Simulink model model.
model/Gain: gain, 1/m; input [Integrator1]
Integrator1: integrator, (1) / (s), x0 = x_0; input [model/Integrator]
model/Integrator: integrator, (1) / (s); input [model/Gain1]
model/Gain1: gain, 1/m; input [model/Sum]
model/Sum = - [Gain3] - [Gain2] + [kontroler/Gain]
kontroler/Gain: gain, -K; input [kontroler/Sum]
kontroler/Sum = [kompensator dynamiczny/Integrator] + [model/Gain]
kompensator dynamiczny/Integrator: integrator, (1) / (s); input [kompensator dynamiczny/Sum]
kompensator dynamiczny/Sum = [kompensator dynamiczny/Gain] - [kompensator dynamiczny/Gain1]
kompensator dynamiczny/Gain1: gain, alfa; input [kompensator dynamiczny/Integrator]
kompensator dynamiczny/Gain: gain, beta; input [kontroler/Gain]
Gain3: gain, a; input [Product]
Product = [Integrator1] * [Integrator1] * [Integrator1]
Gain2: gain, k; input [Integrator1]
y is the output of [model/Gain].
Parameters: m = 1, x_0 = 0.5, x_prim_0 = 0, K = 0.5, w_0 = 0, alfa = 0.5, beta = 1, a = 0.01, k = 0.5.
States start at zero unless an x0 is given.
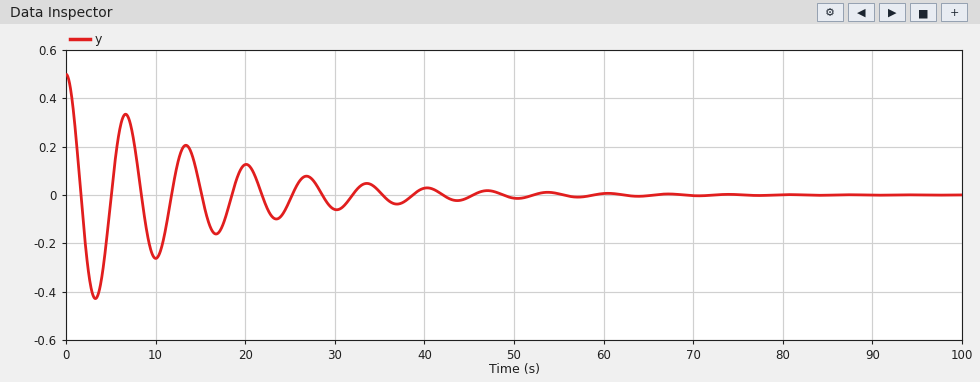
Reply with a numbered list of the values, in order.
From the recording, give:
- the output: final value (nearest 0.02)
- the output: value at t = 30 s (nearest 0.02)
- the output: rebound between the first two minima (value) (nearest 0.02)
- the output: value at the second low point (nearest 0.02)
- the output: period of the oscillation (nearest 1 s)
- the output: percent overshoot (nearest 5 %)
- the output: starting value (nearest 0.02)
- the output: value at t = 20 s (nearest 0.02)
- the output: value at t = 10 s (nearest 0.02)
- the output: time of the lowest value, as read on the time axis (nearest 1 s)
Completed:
1. 0.00
2. -0.06
3. 0.34
4. -0.26
5. 7 s
6. 85 %
7. 0.50
8. 0.12
9. -0.26
10. 3 s
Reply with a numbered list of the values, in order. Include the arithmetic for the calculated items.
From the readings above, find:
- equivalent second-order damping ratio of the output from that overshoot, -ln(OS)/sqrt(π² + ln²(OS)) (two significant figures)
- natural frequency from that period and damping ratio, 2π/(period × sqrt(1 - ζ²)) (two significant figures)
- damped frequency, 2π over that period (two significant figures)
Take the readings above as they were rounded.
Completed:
1. ln(0.85) = -0.163; 0.163 / sqrt(9.870 + 0.026) = 0.052
2. 2π / (7 × sqrt(1 - 0.052²)) = 0.90 rad/s
3. 2π / 7 = 0.90 rad/s
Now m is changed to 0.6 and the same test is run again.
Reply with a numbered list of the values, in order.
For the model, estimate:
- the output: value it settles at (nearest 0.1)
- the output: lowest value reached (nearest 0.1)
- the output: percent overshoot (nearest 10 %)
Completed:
1. 0.0
2. -0.7
3. 80 %
